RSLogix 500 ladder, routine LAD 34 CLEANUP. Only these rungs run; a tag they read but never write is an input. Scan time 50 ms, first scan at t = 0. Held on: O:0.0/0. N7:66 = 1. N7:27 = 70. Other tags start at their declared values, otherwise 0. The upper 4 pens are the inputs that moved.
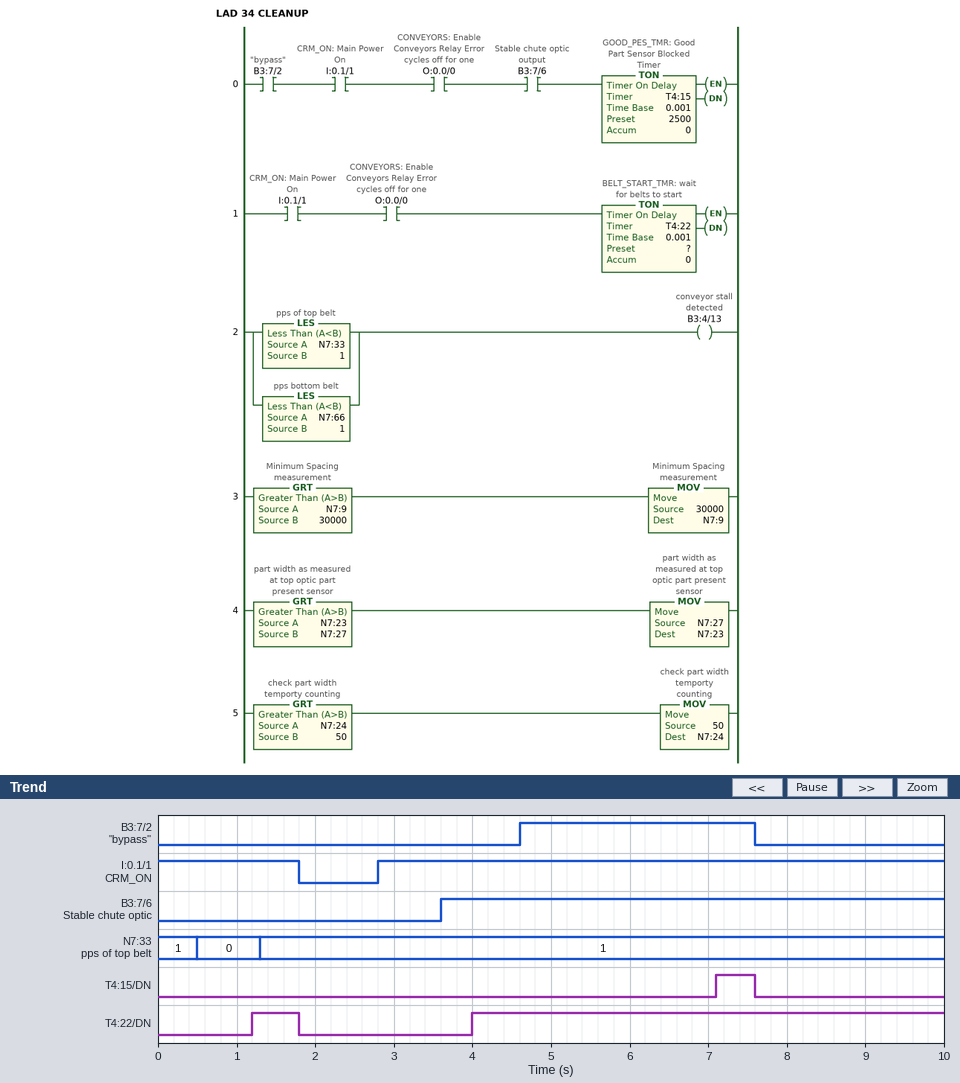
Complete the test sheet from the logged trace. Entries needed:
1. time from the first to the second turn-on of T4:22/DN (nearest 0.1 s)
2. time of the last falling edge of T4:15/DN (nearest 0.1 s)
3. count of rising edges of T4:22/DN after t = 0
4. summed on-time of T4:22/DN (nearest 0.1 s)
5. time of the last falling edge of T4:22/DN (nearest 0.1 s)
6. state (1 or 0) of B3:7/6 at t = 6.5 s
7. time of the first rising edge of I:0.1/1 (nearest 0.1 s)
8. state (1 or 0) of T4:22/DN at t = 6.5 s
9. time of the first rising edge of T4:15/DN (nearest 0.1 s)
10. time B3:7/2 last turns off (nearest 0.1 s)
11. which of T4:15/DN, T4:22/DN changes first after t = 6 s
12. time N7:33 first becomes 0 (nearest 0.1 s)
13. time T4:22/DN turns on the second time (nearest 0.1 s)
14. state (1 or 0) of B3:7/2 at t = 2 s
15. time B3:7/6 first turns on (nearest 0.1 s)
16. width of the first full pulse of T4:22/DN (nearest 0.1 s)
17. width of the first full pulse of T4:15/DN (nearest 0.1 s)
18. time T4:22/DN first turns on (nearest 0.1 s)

2.8 s
7.6 s
2
6.6 s
1.8 s
1
2.8 s
1
7.1 s
7.6 s
T4:15/DN
0.5 s
4.0 s
0
3.6 s
0.6 s
0.5 s
1.2 s
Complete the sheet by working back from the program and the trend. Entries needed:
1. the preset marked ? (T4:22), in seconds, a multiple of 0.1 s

1.2 s
